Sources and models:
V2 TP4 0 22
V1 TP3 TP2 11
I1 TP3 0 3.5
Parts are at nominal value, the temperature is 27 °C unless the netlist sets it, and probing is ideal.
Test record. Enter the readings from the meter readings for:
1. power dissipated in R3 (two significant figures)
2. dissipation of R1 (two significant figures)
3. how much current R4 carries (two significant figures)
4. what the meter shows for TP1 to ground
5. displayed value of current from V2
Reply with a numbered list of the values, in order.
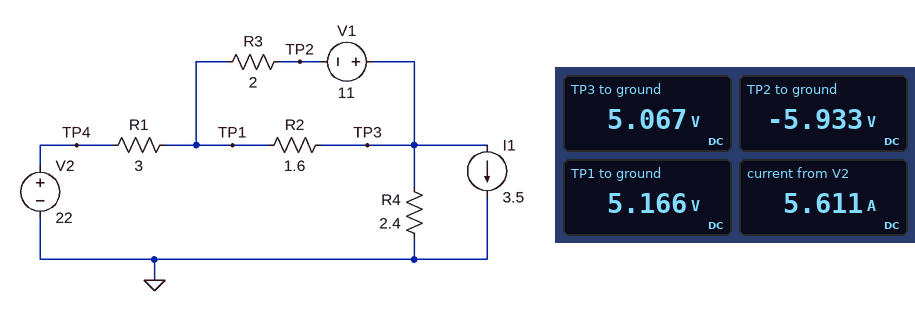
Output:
1. 62 W
2. 94 W
3. 2.1 A
4. 5.166 V
5. 5.611 A
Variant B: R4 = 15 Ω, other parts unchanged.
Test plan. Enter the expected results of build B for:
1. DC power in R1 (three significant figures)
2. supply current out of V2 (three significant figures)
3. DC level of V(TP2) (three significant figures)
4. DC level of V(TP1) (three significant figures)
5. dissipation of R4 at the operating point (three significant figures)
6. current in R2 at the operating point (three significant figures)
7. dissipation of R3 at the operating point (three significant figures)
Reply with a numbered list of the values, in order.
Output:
1. 53.0 W
2. 4.20 A
3. -456 mV
4. 9.39 V
5. 7.41 W
6. 721 mA
7. 48.5 W
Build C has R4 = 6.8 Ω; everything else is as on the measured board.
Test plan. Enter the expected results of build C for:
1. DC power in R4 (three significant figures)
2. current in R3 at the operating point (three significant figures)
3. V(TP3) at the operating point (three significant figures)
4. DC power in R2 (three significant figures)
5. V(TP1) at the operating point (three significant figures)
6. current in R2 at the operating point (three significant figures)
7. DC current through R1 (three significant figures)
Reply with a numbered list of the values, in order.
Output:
1. 10.5 W
2. 5.16 A
3. 8.45 V
4. 284 mW
5. 7.77 V
6. 421 mA
7. 4.74 A
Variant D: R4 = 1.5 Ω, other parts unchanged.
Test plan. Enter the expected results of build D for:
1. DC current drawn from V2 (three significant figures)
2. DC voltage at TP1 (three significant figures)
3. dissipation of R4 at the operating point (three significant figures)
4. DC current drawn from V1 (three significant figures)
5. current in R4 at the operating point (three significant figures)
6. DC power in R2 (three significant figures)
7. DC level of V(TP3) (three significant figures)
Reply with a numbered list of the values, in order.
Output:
1. 5.96 A
2. 4.11 V
3. 9.11 W
4. 5.71 A
5. 2.46 A
6. 106 mW
7. 3.70 V
